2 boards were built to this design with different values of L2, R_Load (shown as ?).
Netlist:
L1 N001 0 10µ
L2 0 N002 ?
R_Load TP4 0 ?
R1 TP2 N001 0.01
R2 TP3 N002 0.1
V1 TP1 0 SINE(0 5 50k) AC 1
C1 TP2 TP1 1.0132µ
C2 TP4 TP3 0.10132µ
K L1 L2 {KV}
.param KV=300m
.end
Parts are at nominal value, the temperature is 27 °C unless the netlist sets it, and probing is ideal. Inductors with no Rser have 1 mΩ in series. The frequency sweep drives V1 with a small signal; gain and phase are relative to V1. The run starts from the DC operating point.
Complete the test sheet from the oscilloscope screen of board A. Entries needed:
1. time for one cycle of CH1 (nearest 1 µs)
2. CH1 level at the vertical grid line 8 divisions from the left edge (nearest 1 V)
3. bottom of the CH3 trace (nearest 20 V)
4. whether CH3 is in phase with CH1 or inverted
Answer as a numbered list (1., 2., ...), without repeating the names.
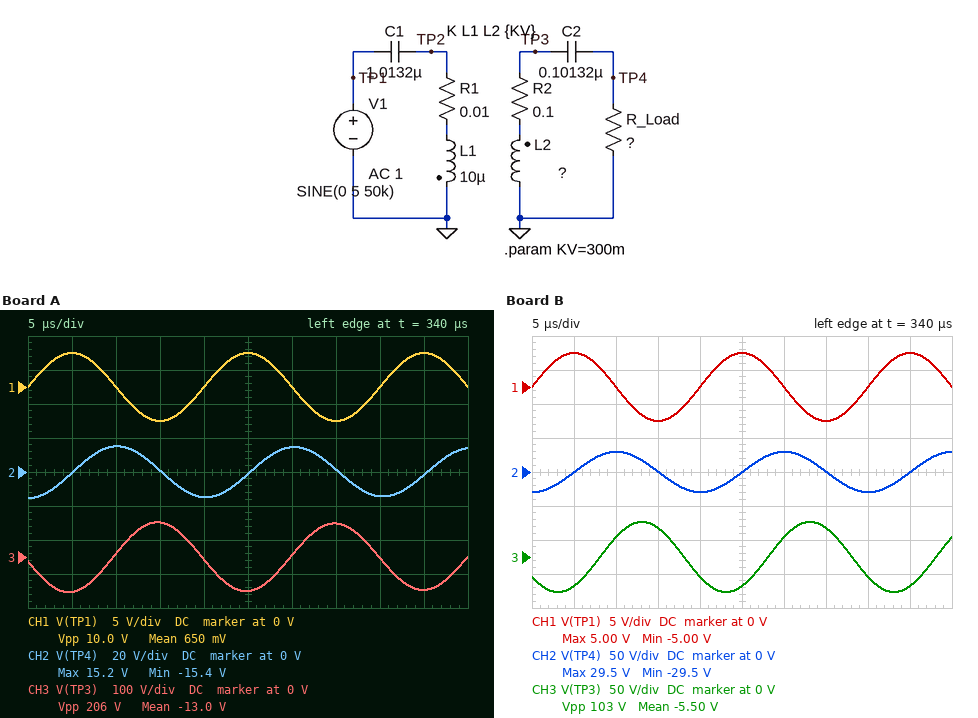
1. 20 µs
2. 0 V
3. -100 V
4. inverted
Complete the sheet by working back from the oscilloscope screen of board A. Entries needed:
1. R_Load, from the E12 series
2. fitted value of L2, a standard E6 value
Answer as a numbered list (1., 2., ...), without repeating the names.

1. 4.7 Ω
2. 47 µH
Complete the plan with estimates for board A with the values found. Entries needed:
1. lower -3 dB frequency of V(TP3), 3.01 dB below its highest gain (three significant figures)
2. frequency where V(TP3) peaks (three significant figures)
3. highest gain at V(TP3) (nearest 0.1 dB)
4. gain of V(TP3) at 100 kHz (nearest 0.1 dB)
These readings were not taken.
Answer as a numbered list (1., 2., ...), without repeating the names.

1. 48.0 kHz
2. 48.4 kHz
3. 34.6 dB
4. 2.0 dB
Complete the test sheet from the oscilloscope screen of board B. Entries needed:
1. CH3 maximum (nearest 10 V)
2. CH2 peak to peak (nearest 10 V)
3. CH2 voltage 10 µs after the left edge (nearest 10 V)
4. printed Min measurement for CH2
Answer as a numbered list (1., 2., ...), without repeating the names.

1. 50 V
2. 60 V
3. 30 V
4. -29.5 V
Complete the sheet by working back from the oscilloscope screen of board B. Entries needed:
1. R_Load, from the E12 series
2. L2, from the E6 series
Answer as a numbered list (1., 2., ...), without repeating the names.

1. 22 Ω
2. 150 µH
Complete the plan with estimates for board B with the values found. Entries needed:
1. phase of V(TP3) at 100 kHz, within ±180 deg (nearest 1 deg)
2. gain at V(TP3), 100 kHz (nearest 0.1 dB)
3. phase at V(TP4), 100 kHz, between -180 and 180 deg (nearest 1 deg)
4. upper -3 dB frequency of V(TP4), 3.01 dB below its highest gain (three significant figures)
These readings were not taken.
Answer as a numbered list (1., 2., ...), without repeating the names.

1. 73 deg
2. -4.6 dB
3. 108 deg
4. 56.4 kHz
